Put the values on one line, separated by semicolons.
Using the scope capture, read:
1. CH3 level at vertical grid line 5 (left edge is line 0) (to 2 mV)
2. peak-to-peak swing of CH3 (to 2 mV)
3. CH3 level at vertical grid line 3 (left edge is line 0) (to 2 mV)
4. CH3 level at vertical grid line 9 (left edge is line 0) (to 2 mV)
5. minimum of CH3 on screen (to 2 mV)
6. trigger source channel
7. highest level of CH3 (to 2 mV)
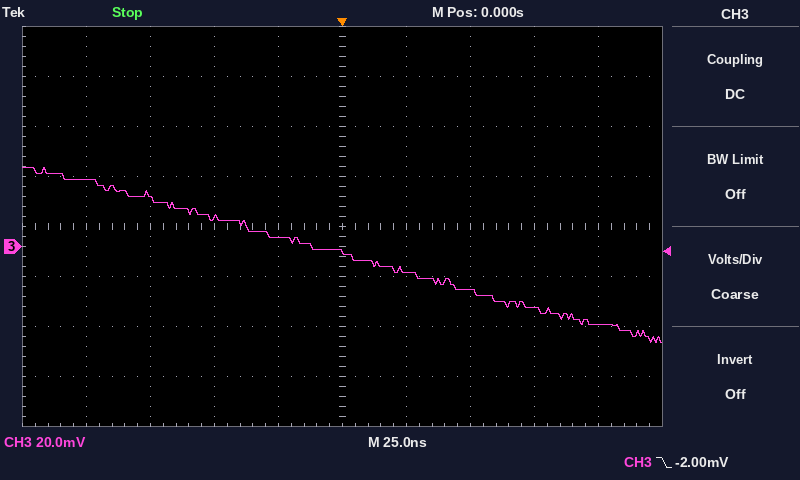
-2 mV; 70 mV; 12 mV; -32 mV; -38 mV; CH3; 32 mV
